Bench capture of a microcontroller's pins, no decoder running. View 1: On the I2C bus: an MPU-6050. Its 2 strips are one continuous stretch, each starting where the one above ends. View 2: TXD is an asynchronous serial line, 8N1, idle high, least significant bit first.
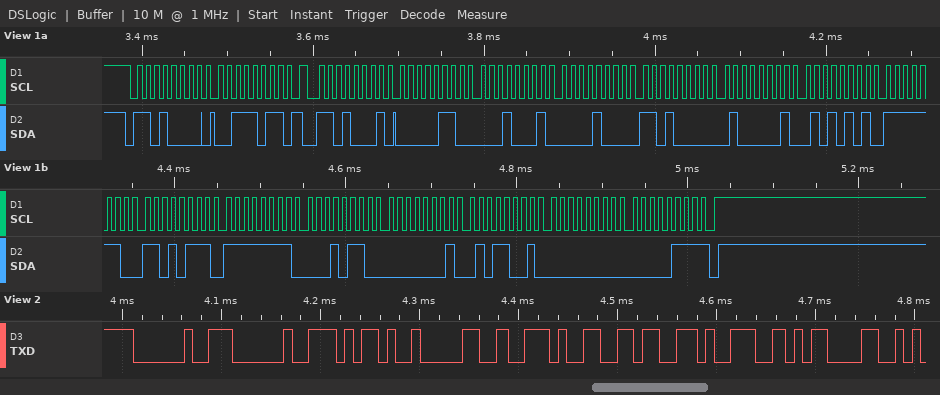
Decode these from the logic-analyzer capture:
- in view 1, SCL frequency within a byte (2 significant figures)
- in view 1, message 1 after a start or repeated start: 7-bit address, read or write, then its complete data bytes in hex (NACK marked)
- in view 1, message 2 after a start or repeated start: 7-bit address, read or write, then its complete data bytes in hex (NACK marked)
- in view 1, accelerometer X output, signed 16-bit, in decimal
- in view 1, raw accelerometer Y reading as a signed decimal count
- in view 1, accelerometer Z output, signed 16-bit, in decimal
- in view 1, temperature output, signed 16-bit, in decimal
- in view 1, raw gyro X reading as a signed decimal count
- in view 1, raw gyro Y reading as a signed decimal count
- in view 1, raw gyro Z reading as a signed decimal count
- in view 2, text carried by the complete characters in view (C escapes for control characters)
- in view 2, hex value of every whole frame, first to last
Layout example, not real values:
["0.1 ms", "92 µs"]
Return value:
["100 kHz", "0x68 write: 3B", "0x68 read: 06 11 08 D0 41 55 FE D7 FF 16 01 59 00 07 NACK", "1553", "2256", "16725", "-297", "-234", "345", "7", "\"  -0.69\\r\"", "0x20 0x20 0x2D 0x30 0x2E 0x36 0x39 0x0D"]
